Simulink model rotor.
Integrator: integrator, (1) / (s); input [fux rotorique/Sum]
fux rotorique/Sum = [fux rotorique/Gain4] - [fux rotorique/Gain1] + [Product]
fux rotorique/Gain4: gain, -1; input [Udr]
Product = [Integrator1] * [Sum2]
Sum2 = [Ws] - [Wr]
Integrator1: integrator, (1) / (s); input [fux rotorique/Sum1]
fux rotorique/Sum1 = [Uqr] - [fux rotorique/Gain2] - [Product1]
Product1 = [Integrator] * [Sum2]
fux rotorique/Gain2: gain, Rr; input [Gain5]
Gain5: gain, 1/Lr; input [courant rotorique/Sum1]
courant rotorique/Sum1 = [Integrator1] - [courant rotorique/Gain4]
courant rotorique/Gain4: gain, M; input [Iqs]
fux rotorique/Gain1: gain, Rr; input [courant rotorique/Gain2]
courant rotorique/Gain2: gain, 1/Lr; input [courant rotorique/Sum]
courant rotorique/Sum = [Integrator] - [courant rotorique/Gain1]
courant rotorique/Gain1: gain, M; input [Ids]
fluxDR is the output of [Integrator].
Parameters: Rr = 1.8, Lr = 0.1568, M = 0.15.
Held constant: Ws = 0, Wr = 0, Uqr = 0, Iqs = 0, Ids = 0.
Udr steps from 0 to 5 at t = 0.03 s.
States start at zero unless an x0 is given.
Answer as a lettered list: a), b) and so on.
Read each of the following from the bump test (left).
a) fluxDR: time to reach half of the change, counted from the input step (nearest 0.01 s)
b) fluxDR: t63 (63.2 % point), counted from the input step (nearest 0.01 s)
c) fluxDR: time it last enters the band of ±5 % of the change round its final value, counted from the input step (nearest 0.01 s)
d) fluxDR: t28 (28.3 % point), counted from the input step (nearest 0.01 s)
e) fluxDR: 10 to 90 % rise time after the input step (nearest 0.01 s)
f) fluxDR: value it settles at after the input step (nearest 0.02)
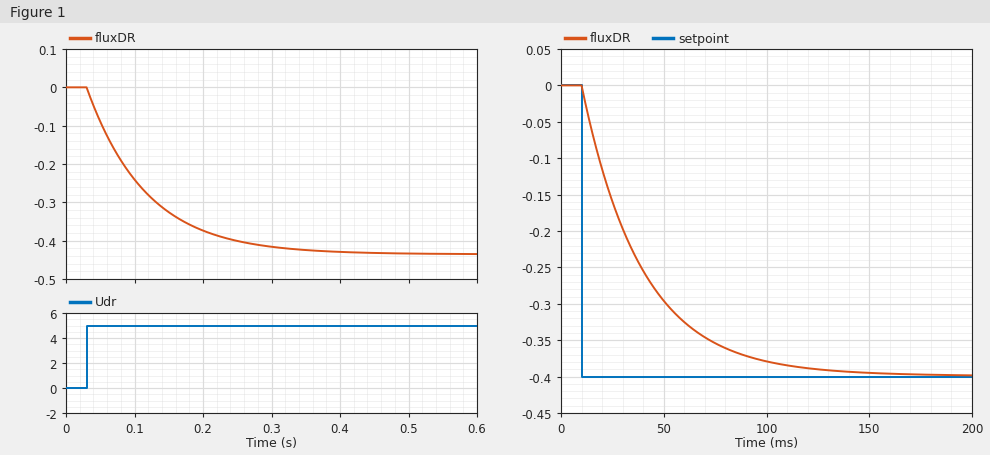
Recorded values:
a) 0.06 s
b) 0.09 s
c) 0.26 s
d) 0.03 s
e) 0.19 s
f) -0.44
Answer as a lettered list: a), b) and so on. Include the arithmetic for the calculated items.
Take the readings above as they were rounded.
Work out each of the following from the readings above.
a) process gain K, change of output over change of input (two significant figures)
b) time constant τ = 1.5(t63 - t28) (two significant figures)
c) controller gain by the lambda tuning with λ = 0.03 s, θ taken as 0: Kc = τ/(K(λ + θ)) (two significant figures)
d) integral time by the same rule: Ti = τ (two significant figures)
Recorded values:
a) (-0.44 - 0) / 5 = -0.088
b) 1.5 × (0.09 - 0.03) = 0.090 s
c) 0.09 / (-0.088 × (0.03 + 0)) = -34
d) 0.090 s
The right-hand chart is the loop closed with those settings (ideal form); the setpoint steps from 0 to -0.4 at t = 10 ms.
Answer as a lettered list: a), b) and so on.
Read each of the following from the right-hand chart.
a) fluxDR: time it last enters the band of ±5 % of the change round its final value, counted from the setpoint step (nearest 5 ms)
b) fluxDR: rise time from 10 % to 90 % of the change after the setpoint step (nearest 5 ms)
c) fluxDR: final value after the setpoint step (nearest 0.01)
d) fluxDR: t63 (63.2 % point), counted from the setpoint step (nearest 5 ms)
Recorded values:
a) 90 ms
b) 65 ms
c) -0.40
d) 30 ms
